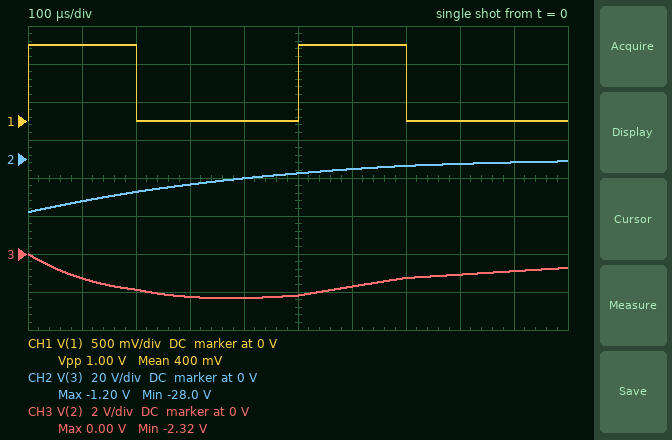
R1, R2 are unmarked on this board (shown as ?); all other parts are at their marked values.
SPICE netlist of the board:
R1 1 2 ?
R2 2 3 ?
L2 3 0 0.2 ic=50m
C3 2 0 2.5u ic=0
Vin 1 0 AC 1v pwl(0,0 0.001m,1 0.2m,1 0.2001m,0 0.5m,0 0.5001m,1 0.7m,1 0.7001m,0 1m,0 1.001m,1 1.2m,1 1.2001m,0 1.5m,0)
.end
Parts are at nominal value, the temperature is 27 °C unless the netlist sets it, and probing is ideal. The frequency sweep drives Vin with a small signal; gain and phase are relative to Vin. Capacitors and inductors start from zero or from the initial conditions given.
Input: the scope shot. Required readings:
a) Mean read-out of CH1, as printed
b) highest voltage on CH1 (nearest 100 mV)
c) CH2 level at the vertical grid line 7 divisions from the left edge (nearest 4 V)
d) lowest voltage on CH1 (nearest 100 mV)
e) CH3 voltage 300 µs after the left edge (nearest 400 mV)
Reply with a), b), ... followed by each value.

a) 400 mV
b) 1.0 V
c) -4 V
d) 0 V
e) -2.4 V
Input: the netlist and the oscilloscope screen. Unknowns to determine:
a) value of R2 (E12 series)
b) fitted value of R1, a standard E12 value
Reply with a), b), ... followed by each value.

a) 560 Ω
b) 150 Ω
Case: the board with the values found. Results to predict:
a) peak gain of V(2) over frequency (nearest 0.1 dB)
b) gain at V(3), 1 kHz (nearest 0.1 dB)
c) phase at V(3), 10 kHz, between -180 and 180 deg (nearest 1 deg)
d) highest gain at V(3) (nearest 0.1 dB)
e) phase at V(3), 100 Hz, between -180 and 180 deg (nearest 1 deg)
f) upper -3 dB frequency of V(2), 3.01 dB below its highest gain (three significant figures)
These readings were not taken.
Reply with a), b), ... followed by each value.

a) -2.1 dB
b) -8.7 dB
c) -85 deg
d) -6.2 dB
e) 69 deg
f) 659 Hz
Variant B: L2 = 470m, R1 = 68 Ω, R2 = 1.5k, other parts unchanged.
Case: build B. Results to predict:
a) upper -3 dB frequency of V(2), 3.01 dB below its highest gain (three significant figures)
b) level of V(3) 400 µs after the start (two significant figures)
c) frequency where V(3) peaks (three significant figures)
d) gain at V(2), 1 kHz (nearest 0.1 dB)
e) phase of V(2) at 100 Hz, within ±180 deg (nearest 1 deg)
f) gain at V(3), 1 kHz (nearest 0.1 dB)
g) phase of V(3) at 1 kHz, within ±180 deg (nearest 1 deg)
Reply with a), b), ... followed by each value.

a) 1.03 kHz
b) -21 V
c) 705 Hz
d) -3.3 dB
e) -5 deg
f) -4.3 dB
g) -19 deg
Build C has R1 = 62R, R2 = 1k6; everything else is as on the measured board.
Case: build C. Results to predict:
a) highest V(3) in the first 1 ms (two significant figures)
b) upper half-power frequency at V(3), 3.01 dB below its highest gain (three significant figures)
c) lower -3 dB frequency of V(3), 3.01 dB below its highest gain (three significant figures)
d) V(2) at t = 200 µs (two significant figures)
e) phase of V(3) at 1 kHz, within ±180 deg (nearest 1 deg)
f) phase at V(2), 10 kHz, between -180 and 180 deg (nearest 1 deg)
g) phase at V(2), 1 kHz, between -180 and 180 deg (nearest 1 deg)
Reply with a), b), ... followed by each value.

a) 67 mV
b) 2.79 kHz
c) 487 Hz
d) -220 mV
e) 9 deg
f) -84 deg
g) -43 deg
